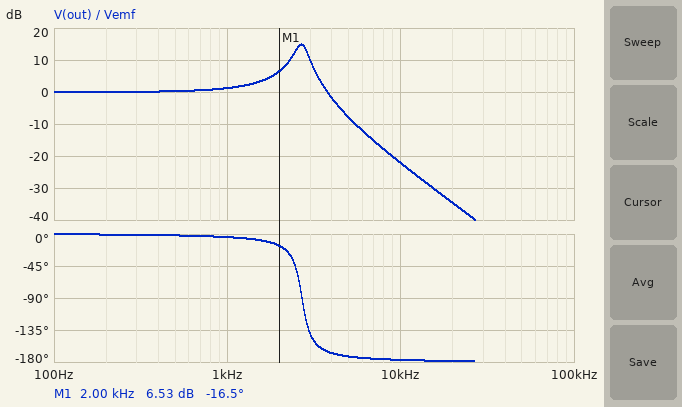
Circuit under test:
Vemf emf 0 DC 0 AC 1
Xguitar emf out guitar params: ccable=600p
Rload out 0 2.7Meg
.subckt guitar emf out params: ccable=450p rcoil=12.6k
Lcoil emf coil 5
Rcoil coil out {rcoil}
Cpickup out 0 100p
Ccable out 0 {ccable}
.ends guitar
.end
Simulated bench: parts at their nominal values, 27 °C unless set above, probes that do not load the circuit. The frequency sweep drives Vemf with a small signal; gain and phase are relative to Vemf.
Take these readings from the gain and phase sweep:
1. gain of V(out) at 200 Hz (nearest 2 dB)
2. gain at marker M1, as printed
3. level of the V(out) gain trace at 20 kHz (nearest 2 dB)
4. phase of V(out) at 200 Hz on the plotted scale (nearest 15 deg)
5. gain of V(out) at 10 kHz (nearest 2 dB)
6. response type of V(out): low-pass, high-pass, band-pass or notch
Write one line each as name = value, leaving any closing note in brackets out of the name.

gain of V(out) at 200 Hz = 0 dB
gain at marker M1, as printed = 6.53 dB
level of the V(out) gain trace at 20 kHz = -34 dB
phase of V(out) at 200 Hz on the plotted scale = 0 deg
gain of V(out) at 10 kHz = -22 dB
response type of V(out): low-pass, high-pass, band-pass or notch = low-pass
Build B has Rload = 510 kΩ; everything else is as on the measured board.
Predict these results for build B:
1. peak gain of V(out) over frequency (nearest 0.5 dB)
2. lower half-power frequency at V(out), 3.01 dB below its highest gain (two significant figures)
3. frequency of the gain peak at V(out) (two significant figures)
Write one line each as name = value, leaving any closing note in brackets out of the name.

peak gain of V(out) over frequency = 10.0 dB
lower half-power frequency at V(out), 3.01 dB below its highest gain = 2.2 kHz
frequency of the gain peak at V(out) = 2.7 kHz
